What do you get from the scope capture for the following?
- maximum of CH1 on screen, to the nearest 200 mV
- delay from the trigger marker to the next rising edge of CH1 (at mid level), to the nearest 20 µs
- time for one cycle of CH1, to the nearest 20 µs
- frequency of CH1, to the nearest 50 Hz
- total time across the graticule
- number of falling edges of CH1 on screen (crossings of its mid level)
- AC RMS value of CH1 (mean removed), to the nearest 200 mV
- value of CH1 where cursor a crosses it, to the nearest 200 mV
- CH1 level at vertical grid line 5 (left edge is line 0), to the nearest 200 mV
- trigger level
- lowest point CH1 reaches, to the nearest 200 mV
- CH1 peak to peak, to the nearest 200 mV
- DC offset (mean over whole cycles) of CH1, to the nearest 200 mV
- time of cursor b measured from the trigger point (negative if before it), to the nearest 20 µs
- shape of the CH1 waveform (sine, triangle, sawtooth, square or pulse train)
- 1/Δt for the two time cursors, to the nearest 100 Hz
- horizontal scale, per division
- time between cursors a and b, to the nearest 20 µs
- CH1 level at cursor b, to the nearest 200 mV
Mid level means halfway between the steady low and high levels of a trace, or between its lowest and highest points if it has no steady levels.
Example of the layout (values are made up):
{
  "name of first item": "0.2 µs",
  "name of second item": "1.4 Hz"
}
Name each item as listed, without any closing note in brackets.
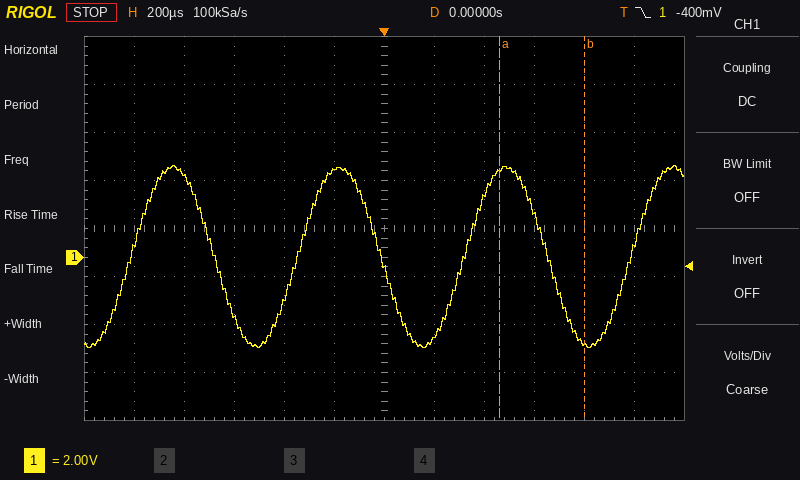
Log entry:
{
  "maximum of CH1 on screen, to the nearest 200 mV": "3.8 V",
  "delay from the trigger marker to the next rising edge of CH1 (at mid level), to the nearest 20 µs": "320 µs",
  "time for one cycle of CH1, to the nearest 20 µs": "660 µs",
  "frequency of CH1, to the nearest 50 Hz": "1.50 kHz",
  "total time across the graticule": "2.4 ms",
  "number of falling edges of CH1 on screen": "3",
  "AC RMS value of CH1 (mean removed), to the nearest 200 mV": "2.6 V",
  "value of CH1 where cursor a crosses it, to the nearest 200 mV": "3.6 V",
  "CH1 level at vertical grid line 5 (left edge is line 0), to the nearest 200 mV": "3.6 V",
  "trigger level": "-400 mV",
  "lowest point CH1 reaches, to the nearest 200 mV": "-3.8 V",
  "CH1 peak to peak, to the nearest 200 mV": "7.6 V",
  "DC offset (mean over whole cycles) of CH1, to the nearest 200 mV": "0.0 V",
  "time of cursor b measured from the trigger point (negative if before it), to the nearest 20 µs": "+800 µs",
  "shape of the CH1 waveform": "sine",
  "1/Δt for the two time cursors, to the nearest 100 Hz": "2.9 kHz",
  "horizontal scale, per division": "200 µs",
  "time between cursors a and b, to the nearest 20 µs": "340 µs",
  "CH1 level at cursor b, to the nearest 200 mV": "-3.6 V"
}
